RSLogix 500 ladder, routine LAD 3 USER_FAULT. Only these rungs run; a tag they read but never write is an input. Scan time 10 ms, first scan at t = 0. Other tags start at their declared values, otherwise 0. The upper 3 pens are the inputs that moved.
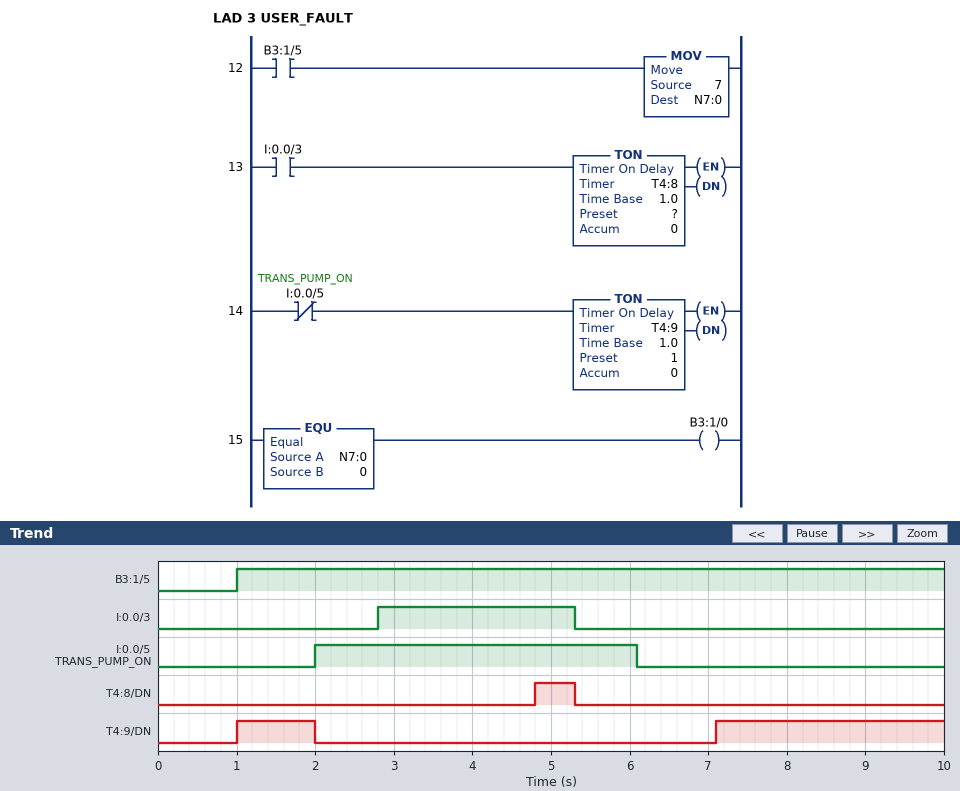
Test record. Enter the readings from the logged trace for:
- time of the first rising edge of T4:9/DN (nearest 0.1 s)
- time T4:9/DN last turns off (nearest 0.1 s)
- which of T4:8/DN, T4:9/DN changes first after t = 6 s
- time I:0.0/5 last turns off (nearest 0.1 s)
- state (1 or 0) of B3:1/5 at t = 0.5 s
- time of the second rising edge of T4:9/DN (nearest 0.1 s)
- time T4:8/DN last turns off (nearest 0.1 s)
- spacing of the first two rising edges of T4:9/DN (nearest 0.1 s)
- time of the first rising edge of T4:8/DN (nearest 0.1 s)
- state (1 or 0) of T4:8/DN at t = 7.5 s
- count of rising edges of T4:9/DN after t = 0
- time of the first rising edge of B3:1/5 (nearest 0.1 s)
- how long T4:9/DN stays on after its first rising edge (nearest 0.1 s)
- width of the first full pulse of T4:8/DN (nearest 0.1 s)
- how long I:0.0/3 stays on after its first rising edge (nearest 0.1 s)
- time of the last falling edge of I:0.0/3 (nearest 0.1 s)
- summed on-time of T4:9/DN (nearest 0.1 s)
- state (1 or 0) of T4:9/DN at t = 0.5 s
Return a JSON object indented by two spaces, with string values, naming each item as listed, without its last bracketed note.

{
  "time of the first rising edge of T4:9/DN": "1.0 s",
  "time T4:9/DN last turns off": "2.0 s",
  "which of T4:8/DN, T4:9/DN changes first after t = 6 s": "T4:9/DN",
  "time I:0.0/5 last turns off": "6.1 s",
  "state (1 or 0) of B3:1/5 at t = 0.5 s": "0",
  "time of the second rising edge of T4:9/DN": "7.1 s",
  "time T4:8/DN last turns off": "5.3 s",
  "spacing of the first two rising edges of T4:9/DN": "6.1 s",
  "time of the first rising edge of T4:8/DN": "4.8 s",
  "state (1 or 0) of T4:8/DN at t = 7.5 s": "0",
  "count of rising edges of T4:9/DN after t = 0": "2",
  "time of the first rising edge of B3:1/5": "1.0 s",
  "how long T4:9/DN stays on after its first rising edge": "1.0 s",
  "width of the first full pulse of T4:8/DN": "0.5 s",
  "how long I:0.0/3 stays on after its first rising edge": "2.5 s",
  "time of the last falling edge of I:0.0/3": "5.3 s",
  "summed on-time of T4:9/DN": "3.9 s",
  "state (1 or 0) of T4:9/DN at t = 0.5 s": "0"
}
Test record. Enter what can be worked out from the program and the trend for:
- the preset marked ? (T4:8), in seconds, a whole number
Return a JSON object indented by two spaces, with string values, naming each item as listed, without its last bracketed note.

{
  "the preset marked ? (T4:8), in seconds, a whole number": "2 s"
}
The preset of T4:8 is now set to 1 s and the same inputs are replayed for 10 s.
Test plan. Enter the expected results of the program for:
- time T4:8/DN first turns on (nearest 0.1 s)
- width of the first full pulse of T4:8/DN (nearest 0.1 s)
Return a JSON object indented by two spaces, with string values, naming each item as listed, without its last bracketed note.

{
  "time T4:8/DN first turns on": "3.8 s",
  "width of the first full pulse of T4:8/DN": "1.5 s"
}
